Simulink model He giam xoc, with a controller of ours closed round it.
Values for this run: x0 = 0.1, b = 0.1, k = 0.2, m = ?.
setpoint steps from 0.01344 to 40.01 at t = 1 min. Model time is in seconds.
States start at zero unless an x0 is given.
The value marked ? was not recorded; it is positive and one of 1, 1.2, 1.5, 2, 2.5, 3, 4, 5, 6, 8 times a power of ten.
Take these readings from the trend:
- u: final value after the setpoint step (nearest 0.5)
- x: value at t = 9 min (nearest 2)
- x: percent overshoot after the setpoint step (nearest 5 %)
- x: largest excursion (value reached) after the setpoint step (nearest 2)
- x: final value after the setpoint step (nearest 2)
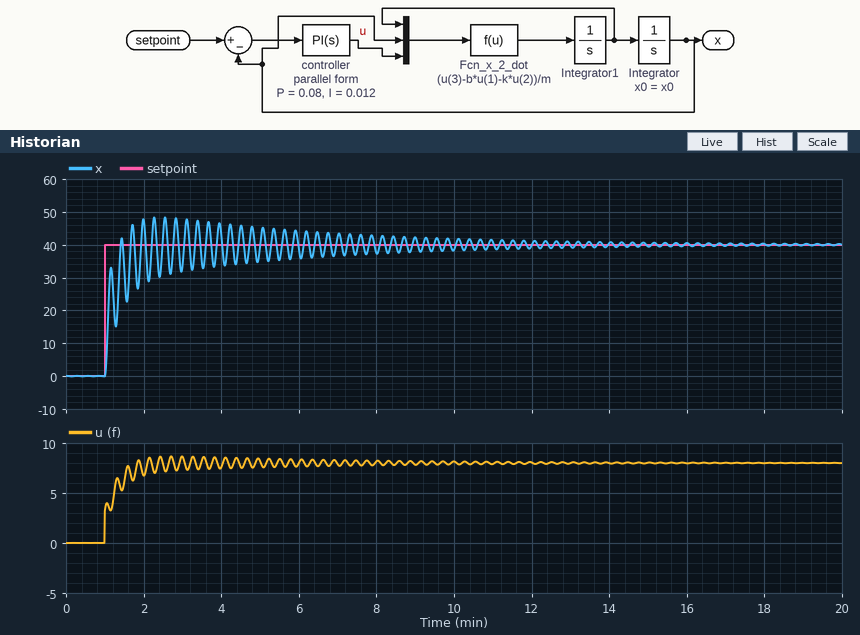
8.0
42
20 %
48
40
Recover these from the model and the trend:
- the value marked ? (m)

2
